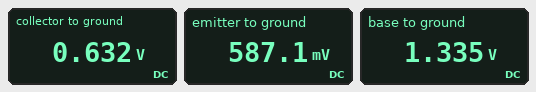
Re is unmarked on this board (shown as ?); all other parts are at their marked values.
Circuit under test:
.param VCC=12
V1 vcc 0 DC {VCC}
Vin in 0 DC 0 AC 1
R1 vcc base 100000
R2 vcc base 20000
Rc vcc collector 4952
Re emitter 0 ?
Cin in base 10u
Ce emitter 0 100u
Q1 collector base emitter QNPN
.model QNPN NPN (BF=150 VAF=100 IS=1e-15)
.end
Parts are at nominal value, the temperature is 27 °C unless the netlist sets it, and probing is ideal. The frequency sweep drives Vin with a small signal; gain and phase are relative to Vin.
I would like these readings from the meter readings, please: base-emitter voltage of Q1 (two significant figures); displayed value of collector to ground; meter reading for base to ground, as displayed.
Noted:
750 mV
0.632 V
1.335 V
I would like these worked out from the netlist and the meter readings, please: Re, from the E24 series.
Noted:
200 Ω
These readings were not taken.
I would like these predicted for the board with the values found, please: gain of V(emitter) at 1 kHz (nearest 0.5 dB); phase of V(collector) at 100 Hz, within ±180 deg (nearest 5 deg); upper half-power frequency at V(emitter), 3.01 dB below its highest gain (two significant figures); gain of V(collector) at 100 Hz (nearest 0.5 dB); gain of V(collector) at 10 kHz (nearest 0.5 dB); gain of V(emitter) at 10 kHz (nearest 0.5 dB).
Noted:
-23.0 dB
-65 deg
1.2 kHz
-15.5 dB
5.5 dB
-39.0 dB
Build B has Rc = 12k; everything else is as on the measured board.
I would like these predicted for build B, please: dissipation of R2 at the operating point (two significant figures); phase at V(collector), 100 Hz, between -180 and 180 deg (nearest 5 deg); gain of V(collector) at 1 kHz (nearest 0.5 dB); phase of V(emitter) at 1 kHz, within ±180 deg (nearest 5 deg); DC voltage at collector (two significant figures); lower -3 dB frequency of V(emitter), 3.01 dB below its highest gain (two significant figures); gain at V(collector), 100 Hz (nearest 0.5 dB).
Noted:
6.0 mW
-55 deg
-4.5 dB
-50 deg
360 mV
7.3 Hz
-18.0 dB
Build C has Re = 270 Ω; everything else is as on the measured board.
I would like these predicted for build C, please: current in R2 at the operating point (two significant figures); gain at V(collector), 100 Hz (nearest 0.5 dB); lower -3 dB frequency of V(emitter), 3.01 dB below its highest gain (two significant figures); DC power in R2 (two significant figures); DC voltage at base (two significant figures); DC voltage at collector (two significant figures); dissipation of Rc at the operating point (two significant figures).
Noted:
520 µA
-15.0 dB
5.7 Hz
5.5 mW
1.5 V
820 mV
25 mW
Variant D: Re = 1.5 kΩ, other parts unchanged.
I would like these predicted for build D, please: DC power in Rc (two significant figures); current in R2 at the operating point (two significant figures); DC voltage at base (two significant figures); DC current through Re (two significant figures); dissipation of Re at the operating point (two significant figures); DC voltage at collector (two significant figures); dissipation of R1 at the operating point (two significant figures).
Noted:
15 mW
400 µA
4.1 V
2.2 mA
7.4 mW
3.4 V
630 µW
